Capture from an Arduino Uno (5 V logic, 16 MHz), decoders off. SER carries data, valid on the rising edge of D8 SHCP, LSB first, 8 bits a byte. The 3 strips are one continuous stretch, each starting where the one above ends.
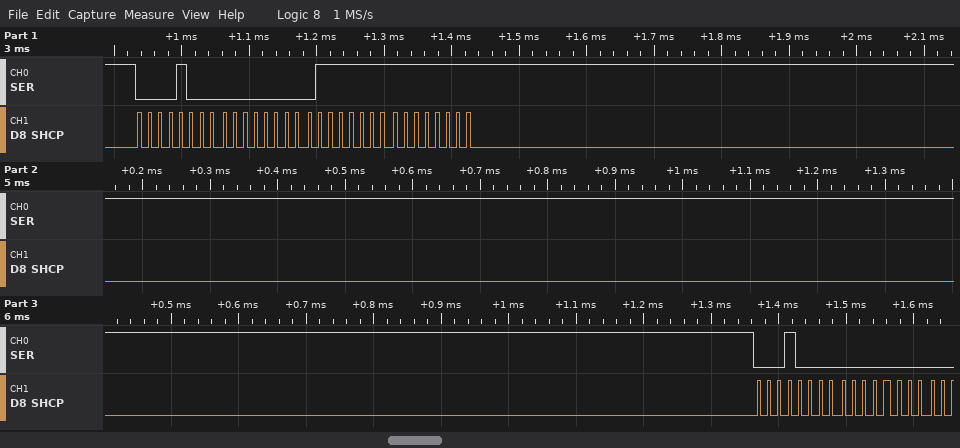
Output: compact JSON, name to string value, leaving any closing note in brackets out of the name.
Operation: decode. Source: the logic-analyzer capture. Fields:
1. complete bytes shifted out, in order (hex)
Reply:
{"complete bytes shifted out, in order": "10 00 FE FF 08 00"}
